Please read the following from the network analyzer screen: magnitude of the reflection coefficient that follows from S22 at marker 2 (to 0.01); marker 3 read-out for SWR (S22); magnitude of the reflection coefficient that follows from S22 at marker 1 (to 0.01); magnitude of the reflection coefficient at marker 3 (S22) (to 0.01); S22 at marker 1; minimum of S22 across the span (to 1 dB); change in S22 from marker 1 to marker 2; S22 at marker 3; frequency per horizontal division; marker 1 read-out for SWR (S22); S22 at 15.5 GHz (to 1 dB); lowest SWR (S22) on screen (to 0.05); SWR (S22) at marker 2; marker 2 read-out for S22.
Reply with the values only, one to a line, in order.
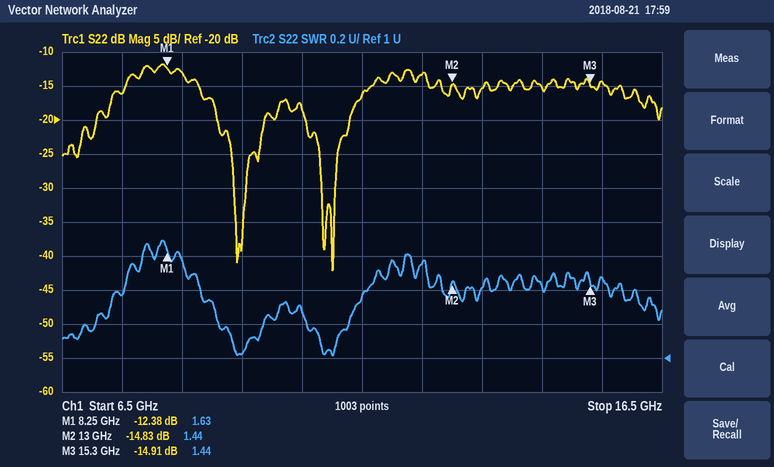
0.18
1.44
0.24
0.18
-12.38 dB
-42 dB
-2.45 dB
-14.91 dB
1 GHz
1.63
-14 dB
1.00
1.44
-14.83 dB
